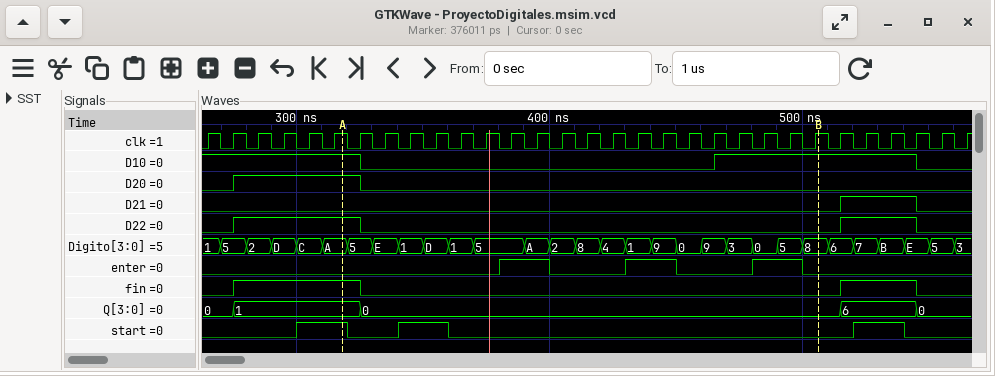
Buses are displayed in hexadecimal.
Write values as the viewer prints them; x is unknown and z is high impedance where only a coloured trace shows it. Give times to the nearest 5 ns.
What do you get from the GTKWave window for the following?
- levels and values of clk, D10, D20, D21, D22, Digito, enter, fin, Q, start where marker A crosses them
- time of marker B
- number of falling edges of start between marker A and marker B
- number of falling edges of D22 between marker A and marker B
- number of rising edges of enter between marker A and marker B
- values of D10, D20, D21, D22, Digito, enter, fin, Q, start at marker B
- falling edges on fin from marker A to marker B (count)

clk=1, D10=1, D20=1, D21=0, D22=1, Digito=A, enter=0, fin=1, Q=1, start=1
505 ns
2
1
3
D10=1, D20=0, D21=0, D22=0, Digito=8, enter=0, fin=0, Q=0, start=0
1
